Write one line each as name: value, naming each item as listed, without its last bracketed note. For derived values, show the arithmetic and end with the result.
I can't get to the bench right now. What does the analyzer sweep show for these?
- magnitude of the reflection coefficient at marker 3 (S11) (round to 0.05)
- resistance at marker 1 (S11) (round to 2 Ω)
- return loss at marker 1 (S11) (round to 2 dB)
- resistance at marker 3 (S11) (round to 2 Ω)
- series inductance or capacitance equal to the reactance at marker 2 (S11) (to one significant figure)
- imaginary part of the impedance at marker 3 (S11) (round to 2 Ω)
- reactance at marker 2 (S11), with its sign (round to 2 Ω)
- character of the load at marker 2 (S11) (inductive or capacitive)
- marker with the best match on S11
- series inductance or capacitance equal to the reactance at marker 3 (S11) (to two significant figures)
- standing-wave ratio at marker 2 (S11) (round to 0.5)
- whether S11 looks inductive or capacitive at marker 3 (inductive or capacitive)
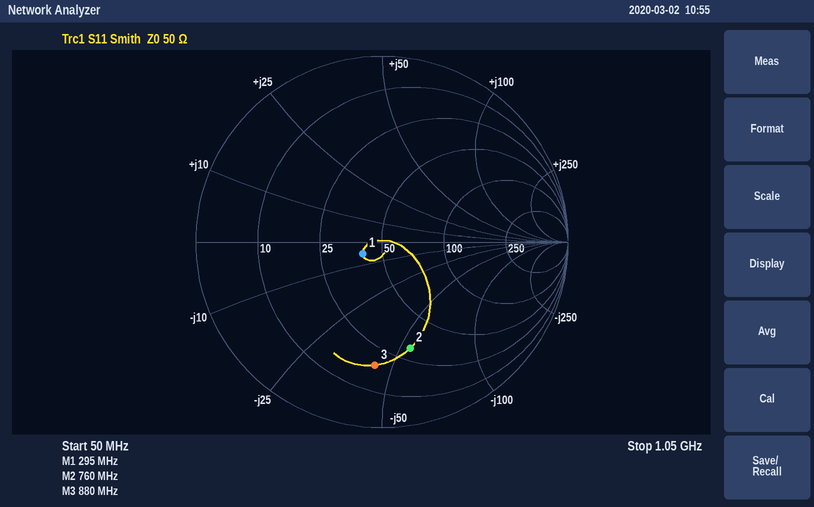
magnitude of the reflection coefficient at marker 3 (S11): 0.65
resistance at marker 1 (S11): 40 Ω
return loss at marker 1 (S11): 18 dB
resistance at marker 3 (S11): 18 Ω
series inductance or capacitance equal to the reactance at marker 2 (S11): C = 1/(2π × 760 MHz × 54 Ω) ≈ 4 pF
imaginary part of the impedance at marker 3 (S11): -44 Ω
reactance at marker 2 (S11), with its sign: -54 Ω
character of the load at marker 2 (S11): capacitive
marker with the best match on S11: marker 1
series inductance or capacitance equal to the reactance at marker 3 (S11): C = 1/(2π × 880 MHz × 44 Ω) ≈ 4.1 pF
standing-wave ratio at marker 2 (S11): 4.0
whether S11 looks inductive or capacitive at marker 3: capacitive
